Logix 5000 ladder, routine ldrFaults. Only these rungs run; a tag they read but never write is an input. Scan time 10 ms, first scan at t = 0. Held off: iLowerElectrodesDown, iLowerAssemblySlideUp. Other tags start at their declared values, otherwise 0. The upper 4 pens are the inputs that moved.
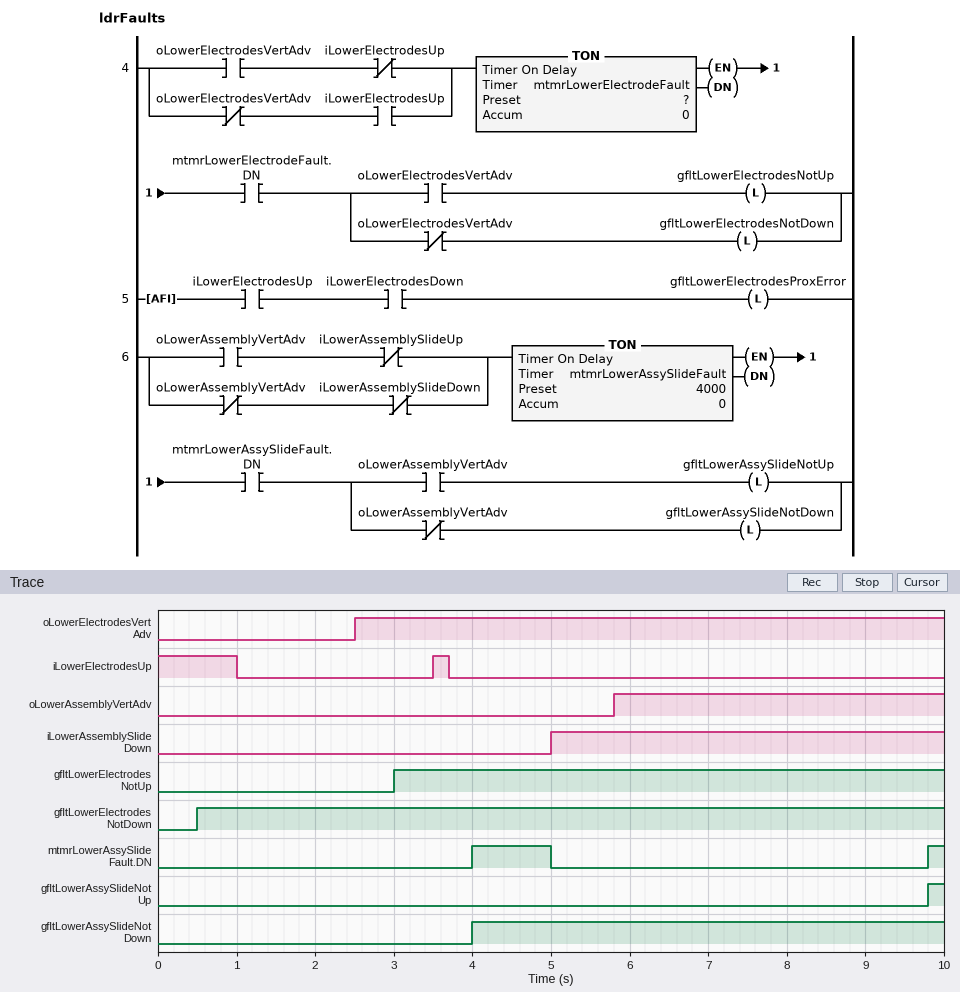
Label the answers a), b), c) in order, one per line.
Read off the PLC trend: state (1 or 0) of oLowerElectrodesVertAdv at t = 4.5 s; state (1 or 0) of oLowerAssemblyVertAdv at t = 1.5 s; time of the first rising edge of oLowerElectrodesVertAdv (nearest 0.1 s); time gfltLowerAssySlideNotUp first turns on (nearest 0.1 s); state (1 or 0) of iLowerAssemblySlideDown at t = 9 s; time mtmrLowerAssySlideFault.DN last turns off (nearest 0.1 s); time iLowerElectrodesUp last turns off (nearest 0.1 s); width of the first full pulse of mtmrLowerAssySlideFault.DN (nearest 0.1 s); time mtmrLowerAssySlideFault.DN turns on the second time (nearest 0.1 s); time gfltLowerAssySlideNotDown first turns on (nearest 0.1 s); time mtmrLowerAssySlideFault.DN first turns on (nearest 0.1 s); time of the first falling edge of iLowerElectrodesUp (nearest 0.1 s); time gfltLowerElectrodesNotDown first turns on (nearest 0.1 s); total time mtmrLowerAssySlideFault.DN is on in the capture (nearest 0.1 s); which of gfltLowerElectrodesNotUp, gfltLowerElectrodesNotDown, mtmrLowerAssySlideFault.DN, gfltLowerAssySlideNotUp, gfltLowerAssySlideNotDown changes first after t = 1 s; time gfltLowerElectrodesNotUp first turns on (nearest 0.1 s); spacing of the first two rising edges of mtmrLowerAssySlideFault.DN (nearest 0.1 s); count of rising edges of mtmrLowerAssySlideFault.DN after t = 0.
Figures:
a) 1
b) 0
c) 2.5 s
d) 9.8 s
e) 1
f) 5.0 s
g) 3.7 s
h) 1.0 s
i) 9.8 s
j) 4.0 s
k) 4.0 s
l) 1.0 s
m) 0.5 s
n) 1.2 s
o) gfltLowerElectrodesNotUp
p) 3.0 s
q) 5.8 s
r) 2
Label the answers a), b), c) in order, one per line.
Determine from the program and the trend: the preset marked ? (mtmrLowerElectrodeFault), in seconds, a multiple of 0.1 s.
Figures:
a) 0.5 s
